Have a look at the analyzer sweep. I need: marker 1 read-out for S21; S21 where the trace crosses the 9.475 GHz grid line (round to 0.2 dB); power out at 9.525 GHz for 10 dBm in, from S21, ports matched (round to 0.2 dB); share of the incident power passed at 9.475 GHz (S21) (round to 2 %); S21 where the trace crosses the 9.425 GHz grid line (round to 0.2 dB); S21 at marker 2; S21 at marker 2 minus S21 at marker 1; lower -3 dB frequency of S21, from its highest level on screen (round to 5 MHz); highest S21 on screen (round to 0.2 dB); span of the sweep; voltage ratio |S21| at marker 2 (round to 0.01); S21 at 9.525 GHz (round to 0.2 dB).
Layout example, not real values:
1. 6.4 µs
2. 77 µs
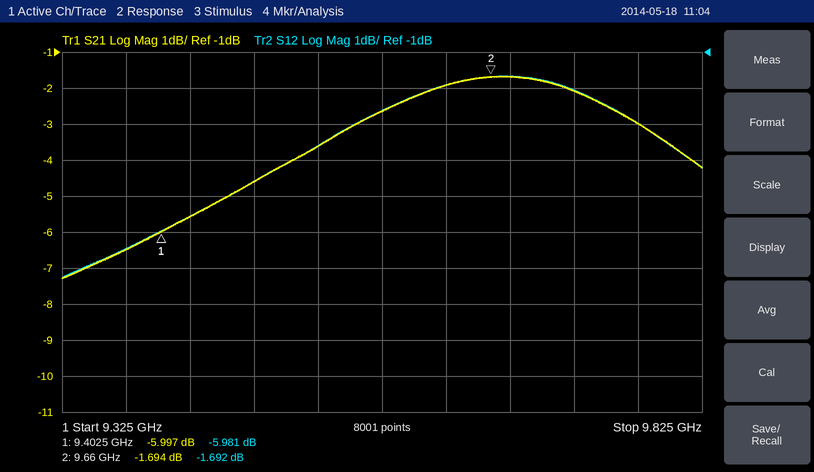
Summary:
1. -5.997 dB
2. -4.6 dB
3. 6.4 dBm
4. 34 %
5. -5.6 dB
6. -1.694 dB
7. 4.303 dB
8. 9.470 GHz
9. -1.6 dB
10. 500 MHz
11. 0.82
12. -3.6 dB
